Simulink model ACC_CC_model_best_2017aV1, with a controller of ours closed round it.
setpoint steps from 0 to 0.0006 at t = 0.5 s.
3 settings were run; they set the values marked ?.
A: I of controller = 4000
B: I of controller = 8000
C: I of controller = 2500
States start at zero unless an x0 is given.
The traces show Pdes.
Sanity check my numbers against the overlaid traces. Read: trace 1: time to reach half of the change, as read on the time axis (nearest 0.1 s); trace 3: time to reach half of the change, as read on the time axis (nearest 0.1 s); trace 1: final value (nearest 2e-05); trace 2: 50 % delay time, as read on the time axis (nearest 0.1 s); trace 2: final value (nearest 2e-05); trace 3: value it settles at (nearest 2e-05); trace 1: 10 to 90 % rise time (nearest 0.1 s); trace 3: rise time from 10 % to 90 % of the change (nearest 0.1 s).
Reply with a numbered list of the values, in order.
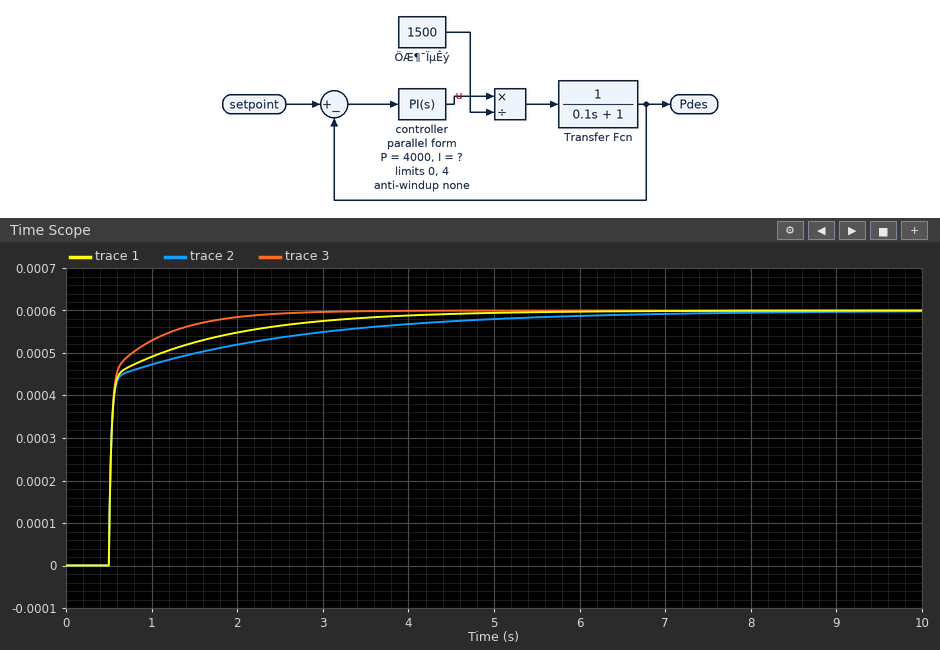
1. 0.5 s
2. 0.5 s
3. 0.00060
4. 0.5 s
5. 0.00060
6. 0.00060
7. 1.3 s
8. 0.6 s
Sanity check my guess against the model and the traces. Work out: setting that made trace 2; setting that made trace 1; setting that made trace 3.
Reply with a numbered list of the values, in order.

1. C
2. A
3. B
